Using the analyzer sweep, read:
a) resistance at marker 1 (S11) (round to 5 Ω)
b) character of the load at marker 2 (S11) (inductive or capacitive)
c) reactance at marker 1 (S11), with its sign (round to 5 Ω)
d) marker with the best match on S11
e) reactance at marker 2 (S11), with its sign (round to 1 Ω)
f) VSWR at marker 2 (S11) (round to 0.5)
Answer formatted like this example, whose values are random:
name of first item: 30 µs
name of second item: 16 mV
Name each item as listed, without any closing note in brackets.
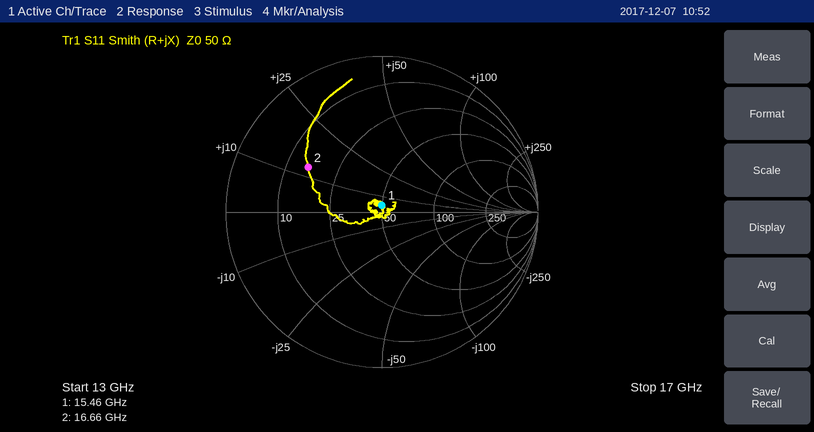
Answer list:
resistance at marker 1 (S11): 50 Ω
character of the load at marker 2 (S11): inductive
reactance at marker 1 (S11), with its sign: +5 Ω
marker with the best match on S11: marker 1
reactance at marker 2 (S11), with its sign: +13 Ω
VSWR at marker 2 (S11): 3.5
